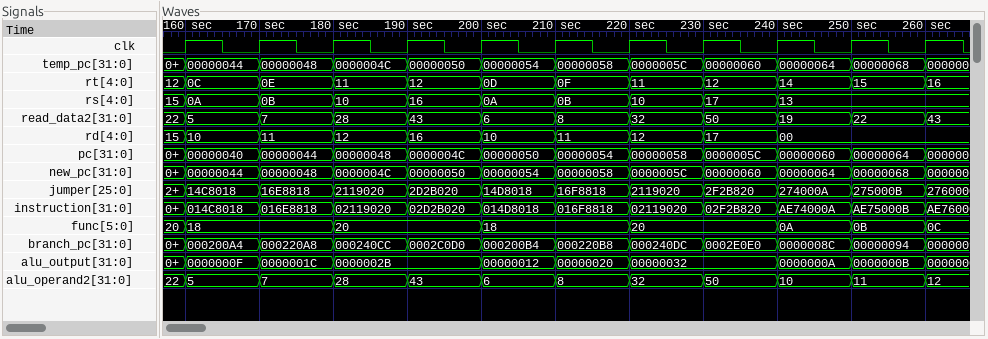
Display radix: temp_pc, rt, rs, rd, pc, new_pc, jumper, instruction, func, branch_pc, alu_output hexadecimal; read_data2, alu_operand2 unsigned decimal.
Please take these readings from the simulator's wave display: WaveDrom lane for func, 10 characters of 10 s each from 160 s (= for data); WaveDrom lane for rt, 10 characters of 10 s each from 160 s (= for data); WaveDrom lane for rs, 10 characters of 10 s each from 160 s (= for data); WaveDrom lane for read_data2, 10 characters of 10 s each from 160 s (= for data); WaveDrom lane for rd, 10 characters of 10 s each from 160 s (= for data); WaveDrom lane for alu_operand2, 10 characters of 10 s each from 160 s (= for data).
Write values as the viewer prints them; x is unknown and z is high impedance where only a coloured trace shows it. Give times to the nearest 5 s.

{name: 'func', wave: '=.=.=.=.==', data: '18 20 18 20 0A 0B'}
{name: 'rt', wave: '==========', data: '0C 0E 11 12 0D 0F 11 12 14 15'}
{name: 'rs', wave: '=========.', data: '0A 0B 10 16 0A 0B 10 17 13'}
{name: 'read_data2', wave: '==========', data: '5 7 28 43 6 8 32 50 19 22'}
{name: 'rd', wave: '=========.', data: '10 11 12 16 10 11 12 17 00'}
{name: 'alu_operand2', wave: '==========', data: '5 7 28 43 6 8 32 50 10 11'}
